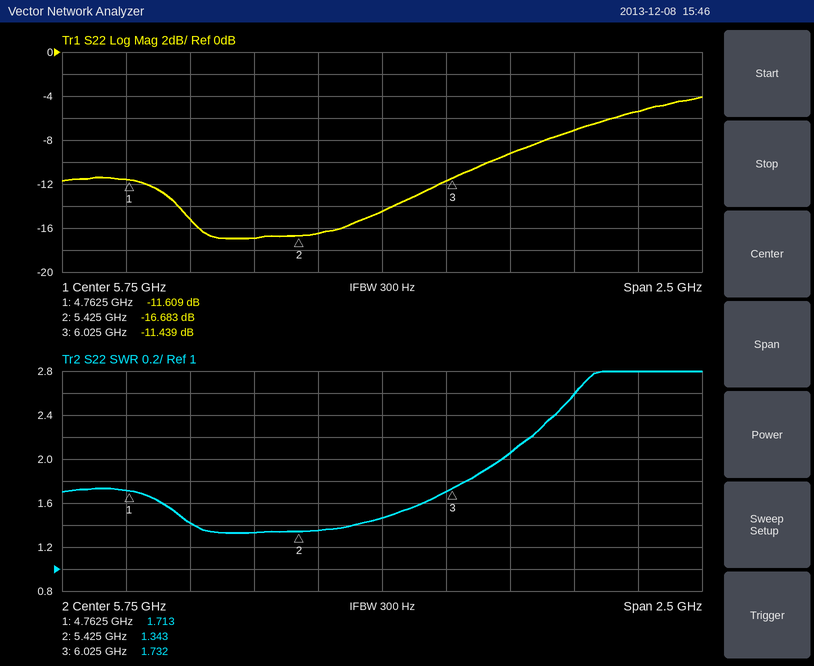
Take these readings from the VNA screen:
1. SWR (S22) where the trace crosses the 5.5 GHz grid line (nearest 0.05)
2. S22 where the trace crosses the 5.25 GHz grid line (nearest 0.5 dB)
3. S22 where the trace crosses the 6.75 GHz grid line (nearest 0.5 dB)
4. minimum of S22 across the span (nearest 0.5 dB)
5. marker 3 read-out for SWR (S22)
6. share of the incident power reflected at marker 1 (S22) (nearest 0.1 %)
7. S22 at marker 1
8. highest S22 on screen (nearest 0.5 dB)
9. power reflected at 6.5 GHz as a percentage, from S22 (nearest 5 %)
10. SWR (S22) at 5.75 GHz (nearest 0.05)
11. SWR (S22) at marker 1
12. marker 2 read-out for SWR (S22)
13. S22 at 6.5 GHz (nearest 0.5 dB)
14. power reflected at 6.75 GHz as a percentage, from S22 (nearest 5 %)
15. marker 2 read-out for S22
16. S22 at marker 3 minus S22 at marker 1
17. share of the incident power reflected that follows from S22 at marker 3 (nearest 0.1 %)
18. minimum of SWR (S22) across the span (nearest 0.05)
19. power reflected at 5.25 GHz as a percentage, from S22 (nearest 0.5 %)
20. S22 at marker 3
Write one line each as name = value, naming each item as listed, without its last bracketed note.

SWR (S22) where the trace crosses the 5.5 GHz grid line = 1.35
S22 where the trace crosses the 5.25 GHz grid line = -17.0 dB
S22 where the trace crosses the 6.75 GHz grid line = -5.5 dB
minimum of S22 across the span = -17.0 dB
marker 3 read-out for SWR = 1.732
share of the incident power reflected at marker 1 (S22) = 6.9 %
S22 at marker 1 = -11.609 dB
highest S22 on screen = -4.0 dB
power reflected at 6.5 GHz as a percentage, from S22 = 20 %
SWR (S22) at 5.75 GHz = 1.45
SWR (S22) at marker 1 = 1.713
marker 2 read-out for SWR = 1.343
S22 at 6.5 GHz = -7.0 dB
power reflected at 6.75 GHz as a percentage, from S22 = 30 %
marker 2 read-out for S22 = -16.683 dB
S22 at marker 3 minus S22 at marker 1 = 0.170 dB
share of the incident power reflected that follows from S22 at marker 3 = 7.2 %
minimum of SWR (S22) across the span = 1.35
power reflected at 5.25 GHz as a percentage, from S22 = 2.0 %
S22 at marker 3 = -11.439 dB
